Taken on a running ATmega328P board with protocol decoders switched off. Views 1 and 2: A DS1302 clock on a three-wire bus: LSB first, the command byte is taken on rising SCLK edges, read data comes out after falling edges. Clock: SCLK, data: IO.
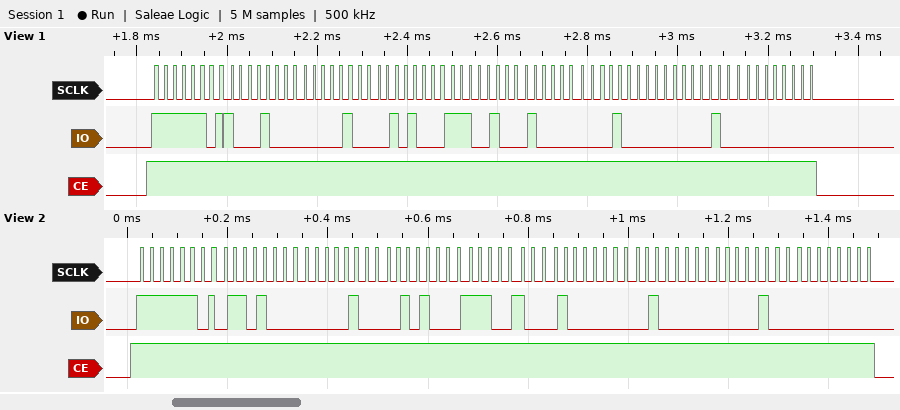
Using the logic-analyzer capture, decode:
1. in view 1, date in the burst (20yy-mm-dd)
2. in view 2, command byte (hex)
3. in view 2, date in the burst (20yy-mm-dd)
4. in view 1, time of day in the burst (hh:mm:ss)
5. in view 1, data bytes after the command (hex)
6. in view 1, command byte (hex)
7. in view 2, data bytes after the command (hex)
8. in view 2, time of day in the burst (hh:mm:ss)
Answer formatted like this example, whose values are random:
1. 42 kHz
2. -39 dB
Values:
1. 2020-02-27
2. 0xBF
3. 2020-02-27
4. 14:20:11
5. 11 20 14 27 02 04 20 00
6. 0xBF
7. 16 20 14 27 02 04 20 00
8. 14:20:16
